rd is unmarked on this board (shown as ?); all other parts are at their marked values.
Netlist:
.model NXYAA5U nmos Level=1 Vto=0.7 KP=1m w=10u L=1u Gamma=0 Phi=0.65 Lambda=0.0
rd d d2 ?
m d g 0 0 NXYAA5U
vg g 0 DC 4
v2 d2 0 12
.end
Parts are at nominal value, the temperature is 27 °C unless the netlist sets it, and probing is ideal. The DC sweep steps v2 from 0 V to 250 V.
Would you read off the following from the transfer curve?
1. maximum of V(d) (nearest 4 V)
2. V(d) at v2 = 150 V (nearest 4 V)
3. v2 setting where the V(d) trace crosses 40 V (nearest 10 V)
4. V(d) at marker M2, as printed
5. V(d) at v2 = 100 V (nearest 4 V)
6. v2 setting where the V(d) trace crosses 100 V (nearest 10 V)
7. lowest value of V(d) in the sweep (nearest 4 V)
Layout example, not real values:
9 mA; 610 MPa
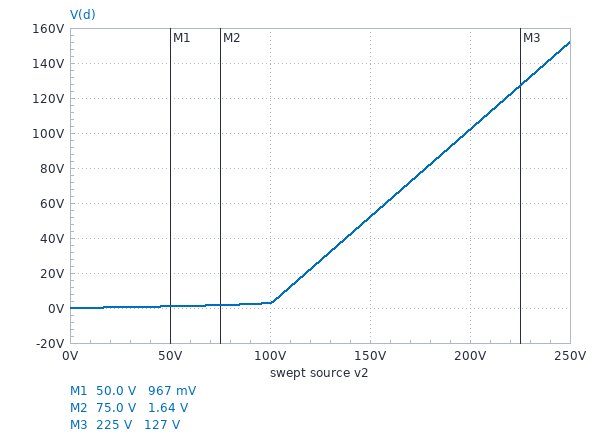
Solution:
152 V; 52 V; 140 V; 1.64 V; 4 V; 200 V; 0 V
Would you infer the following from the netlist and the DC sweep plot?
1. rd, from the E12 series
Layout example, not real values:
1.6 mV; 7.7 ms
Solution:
1.8 kΩ
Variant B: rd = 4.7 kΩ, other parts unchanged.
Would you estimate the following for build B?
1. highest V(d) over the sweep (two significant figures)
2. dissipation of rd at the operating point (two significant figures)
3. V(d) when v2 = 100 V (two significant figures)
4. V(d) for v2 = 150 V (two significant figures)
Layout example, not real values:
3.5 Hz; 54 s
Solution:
2.7 V; 30 mW; 720 mV; 1.2 V
